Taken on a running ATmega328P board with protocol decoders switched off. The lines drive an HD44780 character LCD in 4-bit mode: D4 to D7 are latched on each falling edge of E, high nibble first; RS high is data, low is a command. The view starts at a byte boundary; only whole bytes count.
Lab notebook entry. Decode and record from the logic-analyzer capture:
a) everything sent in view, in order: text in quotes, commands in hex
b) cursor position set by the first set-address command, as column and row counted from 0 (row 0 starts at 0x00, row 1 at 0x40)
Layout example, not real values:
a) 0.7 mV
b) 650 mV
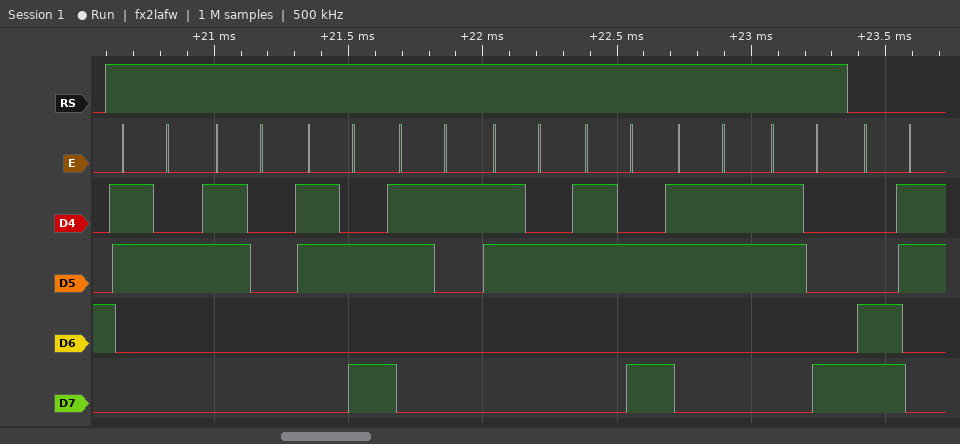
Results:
a) "20:12:38" 0xC3
b) column 3, row 1
